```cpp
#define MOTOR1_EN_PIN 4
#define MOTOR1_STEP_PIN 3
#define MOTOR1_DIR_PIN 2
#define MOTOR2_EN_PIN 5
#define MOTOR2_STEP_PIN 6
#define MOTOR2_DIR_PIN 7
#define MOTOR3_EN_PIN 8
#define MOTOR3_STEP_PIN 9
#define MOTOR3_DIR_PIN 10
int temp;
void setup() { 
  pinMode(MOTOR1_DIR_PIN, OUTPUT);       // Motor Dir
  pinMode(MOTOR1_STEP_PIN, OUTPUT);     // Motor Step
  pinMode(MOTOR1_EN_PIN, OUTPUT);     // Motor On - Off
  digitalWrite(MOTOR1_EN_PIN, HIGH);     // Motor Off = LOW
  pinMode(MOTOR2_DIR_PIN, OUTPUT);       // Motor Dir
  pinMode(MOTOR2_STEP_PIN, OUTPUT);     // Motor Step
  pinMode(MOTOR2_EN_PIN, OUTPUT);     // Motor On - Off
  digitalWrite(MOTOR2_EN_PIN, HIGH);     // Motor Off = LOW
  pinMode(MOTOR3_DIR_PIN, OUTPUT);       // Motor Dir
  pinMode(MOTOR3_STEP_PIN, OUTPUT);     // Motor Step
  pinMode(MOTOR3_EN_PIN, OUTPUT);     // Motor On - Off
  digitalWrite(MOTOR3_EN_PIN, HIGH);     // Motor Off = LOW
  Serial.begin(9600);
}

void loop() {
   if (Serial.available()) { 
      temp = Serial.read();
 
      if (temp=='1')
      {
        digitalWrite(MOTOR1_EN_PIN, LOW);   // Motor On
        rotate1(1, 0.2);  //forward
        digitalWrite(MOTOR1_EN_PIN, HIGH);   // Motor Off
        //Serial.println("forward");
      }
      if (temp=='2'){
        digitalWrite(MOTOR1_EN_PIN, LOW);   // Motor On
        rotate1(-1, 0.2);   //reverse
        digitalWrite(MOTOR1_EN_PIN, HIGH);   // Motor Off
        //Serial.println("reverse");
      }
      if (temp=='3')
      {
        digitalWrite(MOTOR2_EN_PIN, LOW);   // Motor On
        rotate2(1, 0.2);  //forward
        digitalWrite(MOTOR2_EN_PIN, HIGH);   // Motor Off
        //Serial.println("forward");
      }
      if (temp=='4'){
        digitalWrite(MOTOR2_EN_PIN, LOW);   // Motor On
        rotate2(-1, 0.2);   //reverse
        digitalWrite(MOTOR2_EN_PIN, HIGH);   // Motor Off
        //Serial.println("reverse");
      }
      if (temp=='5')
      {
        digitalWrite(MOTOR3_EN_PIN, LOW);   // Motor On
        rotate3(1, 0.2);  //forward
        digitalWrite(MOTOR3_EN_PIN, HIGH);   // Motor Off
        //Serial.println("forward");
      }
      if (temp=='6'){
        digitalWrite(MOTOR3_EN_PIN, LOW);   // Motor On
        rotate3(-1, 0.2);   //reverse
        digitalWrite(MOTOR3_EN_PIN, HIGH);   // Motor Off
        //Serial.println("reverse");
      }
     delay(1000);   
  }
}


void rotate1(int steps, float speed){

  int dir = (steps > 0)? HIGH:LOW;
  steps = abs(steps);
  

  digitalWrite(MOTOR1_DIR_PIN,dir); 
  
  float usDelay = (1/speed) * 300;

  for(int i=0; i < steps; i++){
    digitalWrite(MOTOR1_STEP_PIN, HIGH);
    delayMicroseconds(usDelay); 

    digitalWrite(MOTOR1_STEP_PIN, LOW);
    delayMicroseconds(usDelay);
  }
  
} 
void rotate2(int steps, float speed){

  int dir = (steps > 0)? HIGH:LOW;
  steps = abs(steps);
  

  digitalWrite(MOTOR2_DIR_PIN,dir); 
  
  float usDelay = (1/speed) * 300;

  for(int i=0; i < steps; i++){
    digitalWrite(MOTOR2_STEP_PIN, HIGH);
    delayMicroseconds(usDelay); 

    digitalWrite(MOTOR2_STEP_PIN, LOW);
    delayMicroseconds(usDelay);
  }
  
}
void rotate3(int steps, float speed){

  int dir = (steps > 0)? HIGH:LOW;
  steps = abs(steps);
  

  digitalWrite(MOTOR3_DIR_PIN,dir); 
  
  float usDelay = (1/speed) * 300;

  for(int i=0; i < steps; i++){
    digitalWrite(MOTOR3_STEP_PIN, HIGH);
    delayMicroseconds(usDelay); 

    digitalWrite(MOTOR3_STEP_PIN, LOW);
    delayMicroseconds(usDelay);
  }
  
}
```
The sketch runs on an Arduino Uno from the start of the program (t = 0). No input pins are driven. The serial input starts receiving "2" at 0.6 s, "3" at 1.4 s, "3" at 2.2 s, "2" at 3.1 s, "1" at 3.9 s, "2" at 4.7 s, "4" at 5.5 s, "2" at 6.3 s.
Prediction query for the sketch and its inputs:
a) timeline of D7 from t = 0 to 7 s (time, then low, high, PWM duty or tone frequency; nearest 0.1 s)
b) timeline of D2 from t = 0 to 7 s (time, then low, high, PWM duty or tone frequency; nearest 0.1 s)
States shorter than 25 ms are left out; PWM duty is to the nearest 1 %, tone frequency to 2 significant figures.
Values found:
0 s low; 1.6 s high; 6.6 s low
0 s low; 4.6 s high; 5.6 s low
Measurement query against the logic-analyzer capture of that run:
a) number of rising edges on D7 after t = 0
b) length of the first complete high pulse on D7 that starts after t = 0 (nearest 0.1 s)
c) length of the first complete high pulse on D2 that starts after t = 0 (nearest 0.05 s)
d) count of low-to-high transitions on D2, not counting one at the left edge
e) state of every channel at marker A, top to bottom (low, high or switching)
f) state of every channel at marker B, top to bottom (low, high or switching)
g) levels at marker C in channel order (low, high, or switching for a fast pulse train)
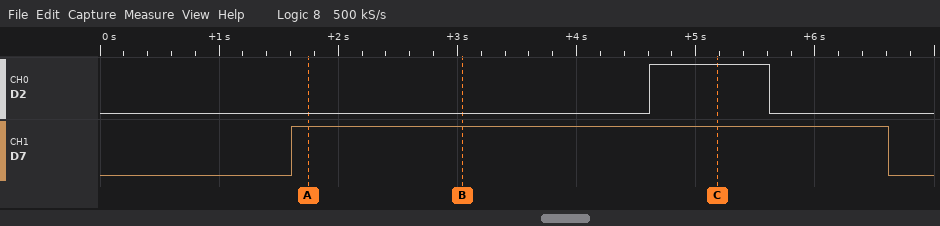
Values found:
1
5.0 s
1.00 s
1
D2 low, D7 high
D2 low, D7 high
D2 high, D7 high
